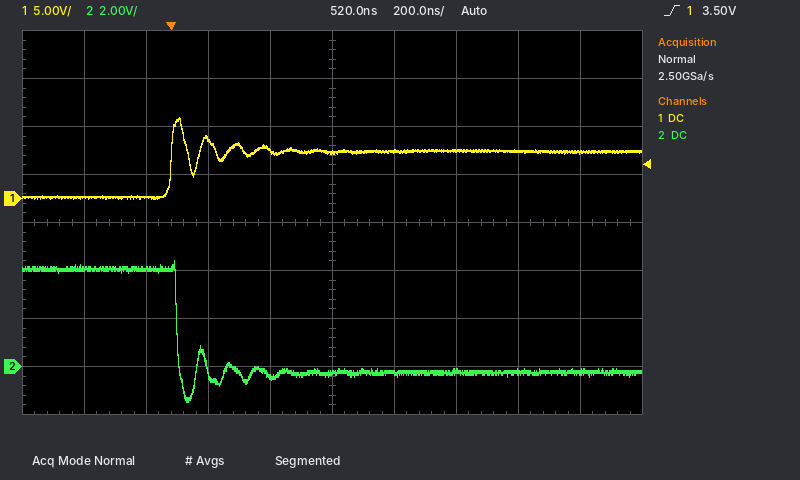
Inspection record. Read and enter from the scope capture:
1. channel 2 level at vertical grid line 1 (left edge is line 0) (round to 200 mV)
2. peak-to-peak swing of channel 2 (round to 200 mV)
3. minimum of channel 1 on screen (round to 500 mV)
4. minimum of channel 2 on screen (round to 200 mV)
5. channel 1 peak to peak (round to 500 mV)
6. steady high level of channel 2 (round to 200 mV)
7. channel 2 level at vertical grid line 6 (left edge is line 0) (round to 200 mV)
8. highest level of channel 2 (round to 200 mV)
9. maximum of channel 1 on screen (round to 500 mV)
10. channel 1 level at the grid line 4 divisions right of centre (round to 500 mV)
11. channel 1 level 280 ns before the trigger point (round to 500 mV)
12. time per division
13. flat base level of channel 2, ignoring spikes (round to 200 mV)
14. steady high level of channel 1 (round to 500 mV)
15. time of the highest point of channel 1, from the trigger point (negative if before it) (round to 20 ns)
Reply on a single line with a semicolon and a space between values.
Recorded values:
4.0 V; 5.8 V; 0.0 V; -1.4 V; 8.5 V; 4.0 V; -200 mV; 4.4 V; 8.5 V; 5.0 V; 0.0 V; 200 ns; -200 mV; 5.0 V; +20 ns
